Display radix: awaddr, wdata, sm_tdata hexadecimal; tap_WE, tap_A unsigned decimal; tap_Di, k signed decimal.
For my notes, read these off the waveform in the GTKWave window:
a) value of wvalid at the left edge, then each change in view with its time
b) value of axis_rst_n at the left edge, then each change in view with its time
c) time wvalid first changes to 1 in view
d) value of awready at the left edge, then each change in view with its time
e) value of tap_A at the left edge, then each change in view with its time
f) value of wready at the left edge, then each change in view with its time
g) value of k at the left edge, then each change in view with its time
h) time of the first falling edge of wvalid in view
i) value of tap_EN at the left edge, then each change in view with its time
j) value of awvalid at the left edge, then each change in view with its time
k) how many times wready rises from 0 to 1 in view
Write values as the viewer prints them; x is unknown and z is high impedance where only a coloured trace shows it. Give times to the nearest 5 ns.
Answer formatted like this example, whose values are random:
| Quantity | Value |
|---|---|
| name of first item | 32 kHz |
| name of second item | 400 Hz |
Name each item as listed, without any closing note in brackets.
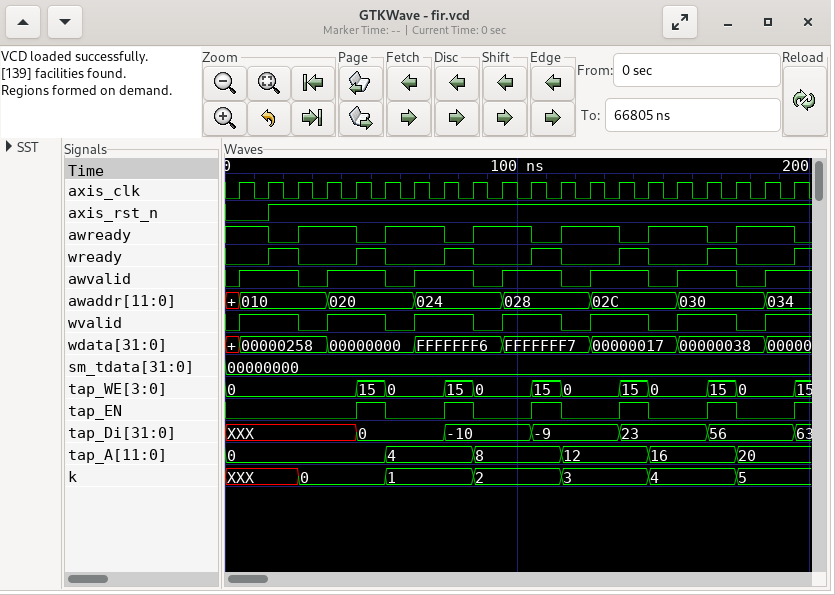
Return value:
| Quantity | Value |
|---|---|
| value of wvalid at the left edge, then each change in view with its time | 0, 1 at 5 ns, 0 at 25 ns, 1 at 35 ns, 0 at 55 ns, 1 at 65 ns, 0 at 85 ns, 1 at 95 ns, 0 at 115 ns, 1 at 125 ns, 0 at 145 ns, 1 at 155 ns, 0 at 175 ns, 1 at 185 ns |
| value of axis_rst_n at the left edge, then each change in view with its time | 0, 1 at 15 ns |
| time wvalid first changes to 1 in view | 5 ns |
| value of awready at the left edge, then each change in view with its time | 1, 0 at 15 ns, 1 at 25 ns, 0 at 45 ns, 1 at 55 ns, 0 at 75 ns, 1 at 85 ns, 0 at 105 ns, 1 at 115 ns, 0 at 135 ns, 1 at 145 ns, 0 at 165 ns, 1 at 175 ns, 0 at 195 ns |
| value of tap_A at the left edge, then each change in view with its time | 0, 4 at 55 ns, 8 at 85 ns, 12 at 115 ns, 16 at 145 ns, 20 at 175 ns |
| value of wready at the left edge, then each change in view with its time | 0, 1 at 15 ns, 0 at 25 ns, 1 at 45 ns, 0 at 55 ns, 1 at 75 ns, 0 at 85 ns, 1 at 105 ns, 0 at 115 ns, 1 at 135 ns, 0 at 145 ns, 1 at 165 ns, 0 at 175 ns, 1 at 195 ns |
| value of k at the left edge, then each change in view with its time | XXX, 0 at 25 ns, 1 at 55 ns, 2 at 85 ns, 3 at 115 ns, 4 at 145 ns, 5 at 175 ns |
| time of the first falling edge of wvalid in view | 25 ns |
| value of tap_EN at the left edge, then each change in view with its time | 0, 1 at 45 ns, 0 at 55 ns, 1 at 75 ns, 0 at 85 ns, 1 at 105 ns, 0 at 115 ns, 1 at 135 ns, 0 at 145 ns, 1 at 165 ns, 0 at 175 ns, 1 at 195 ns |
| value of awvalid at the left edge, then each change in view with its time | 0, 1 at 5 ns, 0 at 25 ns, 1 at 35 ns, 0 at 55 ns, 1 at 65 ns, 0 at 85 ns, 1 at 95 ns, 0 at 115 ns, 1 at 125 ns, 0 at 145 ns, 1 at 155 ns, 0 at 175 ns, 1 at 185 ns |
| how many times wready rises from 0 to 1 in view | 7 |
